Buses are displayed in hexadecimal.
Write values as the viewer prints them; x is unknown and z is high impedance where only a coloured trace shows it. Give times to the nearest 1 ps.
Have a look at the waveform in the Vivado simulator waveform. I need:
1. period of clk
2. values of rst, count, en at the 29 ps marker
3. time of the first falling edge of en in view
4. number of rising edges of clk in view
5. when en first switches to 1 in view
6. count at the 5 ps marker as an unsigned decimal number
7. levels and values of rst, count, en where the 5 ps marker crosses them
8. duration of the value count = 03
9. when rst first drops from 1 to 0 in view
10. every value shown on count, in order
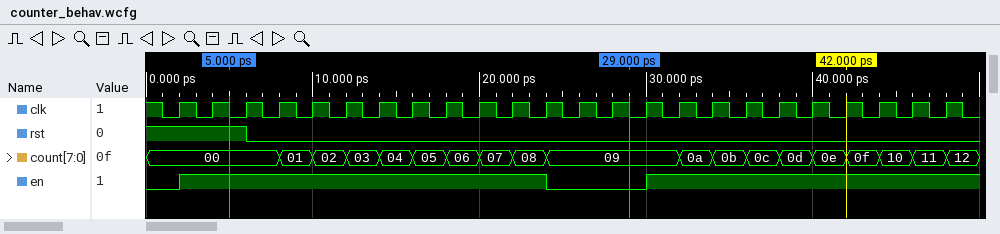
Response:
2 ps
rst=0, count=09, en=0
24 ps
24
2 ps
0
rst=1, count=00, en=1
2 ps
6 ps
00, 01, 02, 03, 04, 05, 06, 07, 08, 09, 0a, 0b, 0c, 0d, 0e, 0f, 10, 11, 12
